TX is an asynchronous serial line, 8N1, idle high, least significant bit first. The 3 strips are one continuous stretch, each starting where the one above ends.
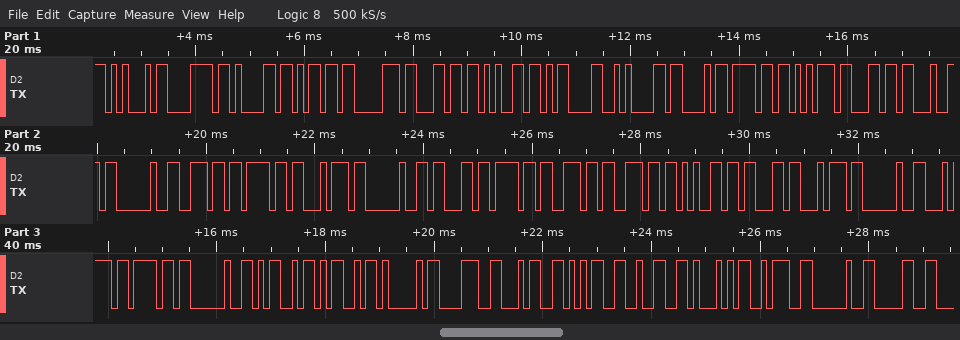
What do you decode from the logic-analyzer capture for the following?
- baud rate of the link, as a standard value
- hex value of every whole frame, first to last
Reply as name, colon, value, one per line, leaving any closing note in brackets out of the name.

baud rate of the link, as a standard value: 9600 baud
hex value of every whole frame, first to last: 45 78 61 6D 70 6C 65 0D 0A 43 6F 75 6C 64 20 6E 6F 74 20 63 6F 6E 6E 65 63 74 20 74 6F 20 4D 4D 41 38 34 35 32 51 3A 20 30
